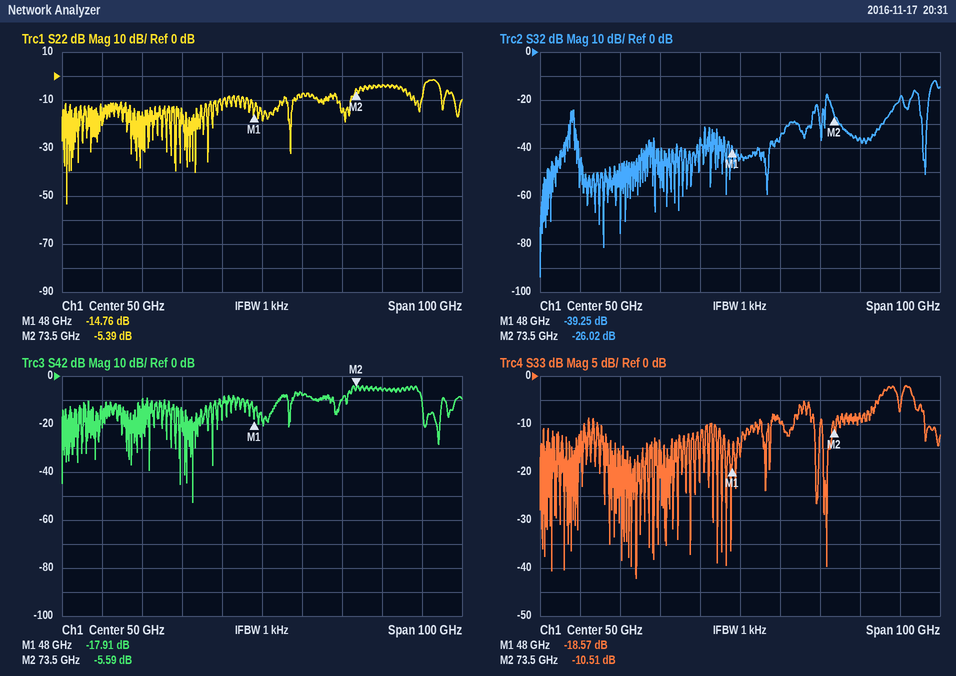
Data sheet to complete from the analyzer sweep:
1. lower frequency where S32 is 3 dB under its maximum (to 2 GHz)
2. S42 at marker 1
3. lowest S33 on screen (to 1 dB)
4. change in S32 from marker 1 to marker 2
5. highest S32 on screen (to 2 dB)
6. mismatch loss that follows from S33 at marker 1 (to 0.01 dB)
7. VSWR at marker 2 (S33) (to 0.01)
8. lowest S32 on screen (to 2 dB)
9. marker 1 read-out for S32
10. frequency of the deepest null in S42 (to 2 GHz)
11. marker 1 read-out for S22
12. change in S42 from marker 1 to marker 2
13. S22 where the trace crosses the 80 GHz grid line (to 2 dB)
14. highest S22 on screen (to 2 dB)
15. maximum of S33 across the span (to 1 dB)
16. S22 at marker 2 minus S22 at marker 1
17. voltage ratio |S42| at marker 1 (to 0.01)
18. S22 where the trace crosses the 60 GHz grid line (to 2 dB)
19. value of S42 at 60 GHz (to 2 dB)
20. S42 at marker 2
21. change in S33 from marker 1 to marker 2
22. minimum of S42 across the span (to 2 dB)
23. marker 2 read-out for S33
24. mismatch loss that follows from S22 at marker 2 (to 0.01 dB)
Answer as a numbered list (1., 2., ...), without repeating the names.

1. 98 GHz
2. -17.91 dB
3. -42 dB
4. 13.23 dB
5. -12 dB
6. 0.06 dB
7. 1.85
8. -94 dB
9. -39.25 dB
10. 32 GHz
11. -14.76 dB
12. 12.32 dB
13. -4 dB
14. -2 dB
15. -2 dB
16. 9.37 dB
17. 0.13
18. -8 dB
19. -8 dB
20. -5.59 dB
21. 8.06 dB
22. -52 dB
23. -10.51 dB
24. 1.48 dB
